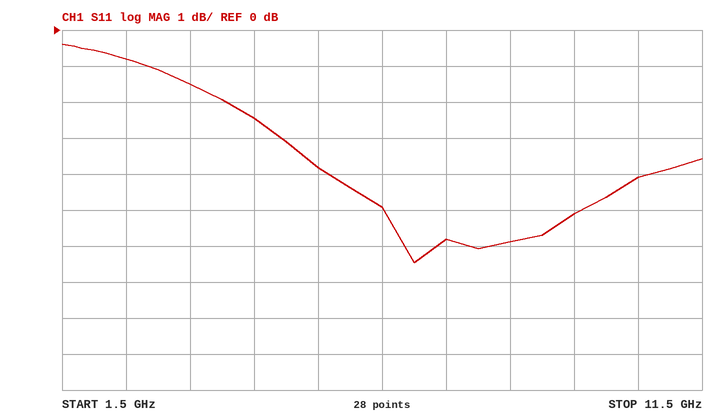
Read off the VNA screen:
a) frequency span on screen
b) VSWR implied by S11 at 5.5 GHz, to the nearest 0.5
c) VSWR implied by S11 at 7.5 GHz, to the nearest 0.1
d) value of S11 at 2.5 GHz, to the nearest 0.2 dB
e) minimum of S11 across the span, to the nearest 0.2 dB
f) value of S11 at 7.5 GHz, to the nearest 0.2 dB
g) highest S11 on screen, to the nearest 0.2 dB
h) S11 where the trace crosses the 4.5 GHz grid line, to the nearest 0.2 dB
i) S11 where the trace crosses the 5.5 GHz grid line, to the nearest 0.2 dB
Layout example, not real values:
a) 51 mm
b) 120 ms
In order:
a) 10 GHz
b) 4.5
c) 3.1
d) -0.8 dB
e) -6.4 dB
f) -5.8 dB
g) -0.4 dB
h) -2.4 dB
i) -3.8 dB
